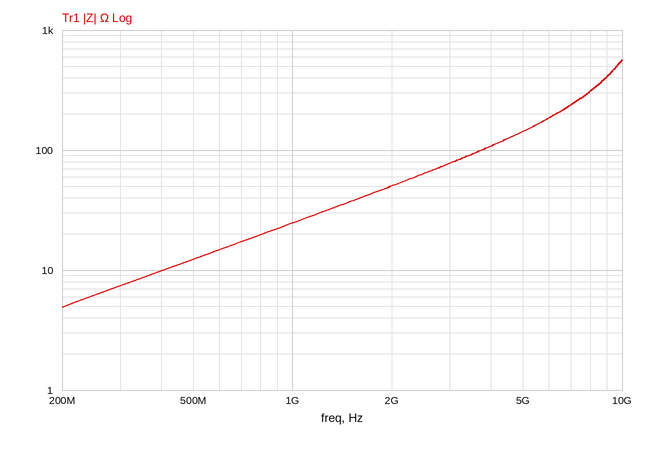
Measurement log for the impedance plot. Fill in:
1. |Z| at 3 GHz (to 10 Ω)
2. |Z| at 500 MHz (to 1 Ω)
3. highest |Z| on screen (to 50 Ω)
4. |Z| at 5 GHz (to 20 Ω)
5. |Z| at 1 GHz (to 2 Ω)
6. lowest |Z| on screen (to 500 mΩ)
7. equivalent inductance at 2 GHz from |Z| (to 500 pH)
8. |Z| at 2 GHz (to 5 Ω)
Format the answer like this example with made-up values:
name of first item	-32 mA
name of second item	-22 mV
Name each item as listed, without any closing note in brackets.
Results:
|Z| at 3 GHz	80 Ω
|Z| at 500 MHz	12 Ω
highest |Z| on screen	550 Ω
|Z| at 5 GHz	140 Ω
|Z| at 1 GHz	24 Ω
lowest |Z| on screen	5.0 Ω
equivalent inductance at 2 GHz from |Z|	4.0 nH
|Z| at 2 GHz	50 Ω
